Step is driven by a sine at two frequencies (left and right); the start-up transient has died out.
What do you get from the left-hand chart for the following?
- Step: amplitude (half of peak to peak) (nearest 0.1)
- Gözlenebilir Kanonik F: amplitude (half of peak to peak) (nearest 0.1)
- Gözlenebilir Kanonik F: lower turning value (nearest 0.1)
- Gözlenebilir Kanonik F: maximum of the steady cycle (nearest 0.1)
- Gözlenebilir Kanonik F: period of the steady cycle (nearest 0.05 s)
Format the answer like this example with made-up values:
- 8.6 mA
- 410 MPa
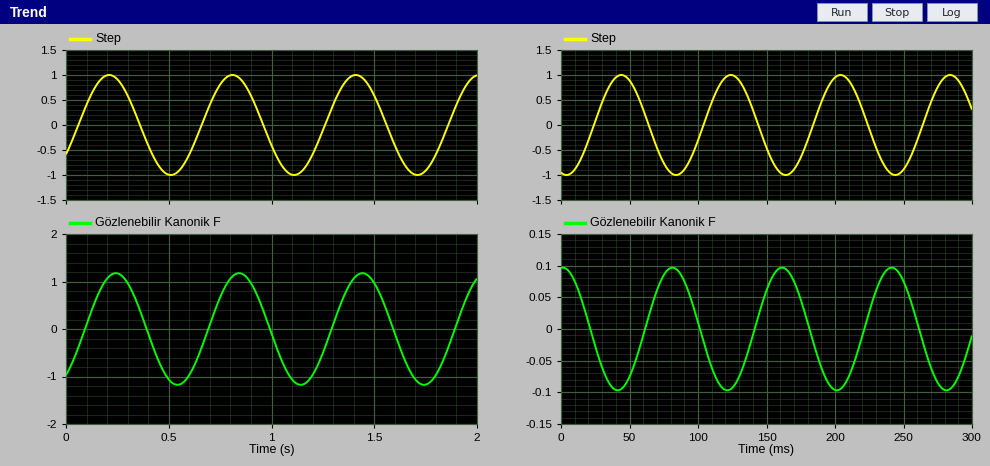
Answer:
- 1.0
- 1.2
- -1.2
- 1.2
- 0.60 s
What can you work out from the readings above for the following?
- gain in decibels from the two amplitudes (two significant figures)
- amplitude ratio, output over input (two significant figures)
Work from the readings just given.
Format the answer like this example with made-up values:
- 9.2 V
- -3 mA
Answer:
- 1.6 dB
- 1.2
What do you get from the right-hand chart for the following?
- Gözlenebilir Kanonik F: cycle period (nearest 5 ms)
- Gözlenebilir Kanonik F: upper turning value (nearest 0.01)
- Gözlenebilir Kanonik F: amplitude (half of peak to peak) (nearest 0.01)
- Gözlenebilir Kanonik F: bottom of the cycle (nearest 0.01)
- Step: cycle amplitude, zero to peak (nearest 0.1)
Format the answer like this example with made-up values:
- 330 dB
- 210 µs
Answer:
- 80 ms
- 0.10
- 0.10
- -0.10
- 1.0
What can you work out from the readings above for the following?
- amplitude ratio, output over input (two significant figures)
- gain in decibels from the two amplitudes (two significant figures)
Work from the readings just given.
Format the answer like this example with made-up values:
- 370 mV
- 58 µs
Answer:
- 0.10
- -20 dB
